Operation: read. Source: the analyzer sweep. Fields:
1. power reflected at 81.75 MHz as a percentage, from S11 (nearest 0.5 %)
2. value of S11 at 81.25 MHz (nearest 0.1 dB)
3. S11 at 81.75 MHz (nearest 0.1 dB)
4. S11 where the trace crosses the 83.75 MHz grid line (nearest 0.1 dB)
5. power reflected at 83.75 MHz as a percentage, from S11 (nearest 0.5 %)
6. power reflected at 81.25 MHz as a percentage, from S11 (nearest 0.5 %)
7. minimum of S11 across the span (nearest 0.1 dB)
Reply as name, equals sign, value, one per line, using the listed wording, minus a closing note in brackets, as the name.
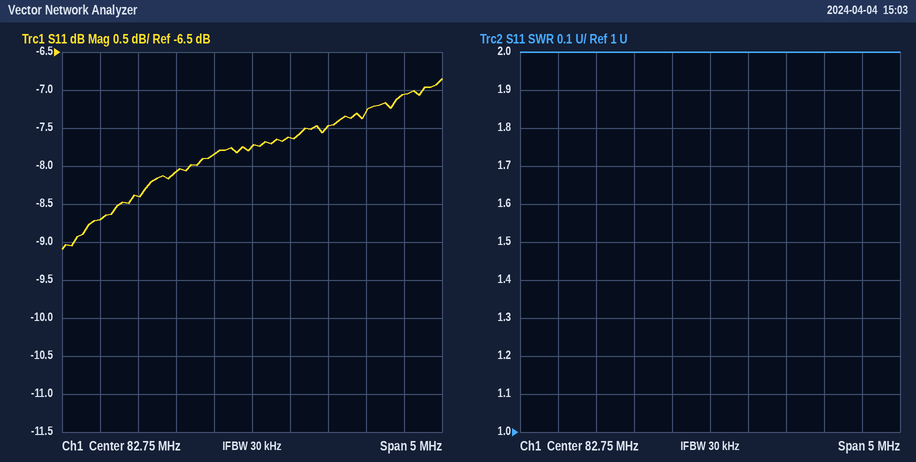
power reflected at 81.75 MHz as a percentage, from S11 = 15.5 %
value of S11 at 81.25 MHz = -8.4 dB
S11 at 81.75 MHz = -8.1 dB
S11 where the trace crosses the 83.75 MHz grid line = -7.5 dB
power reflected at 83.75 MHz as a percentage, from S11 = 18.0 %
power reflected at 81.25 MHz as a percentage, from S11 = 14.5 %
minimum of S11 across the span = -9.1 dB
